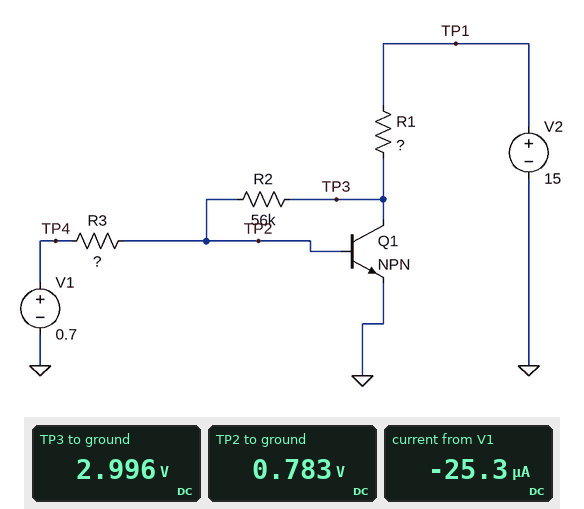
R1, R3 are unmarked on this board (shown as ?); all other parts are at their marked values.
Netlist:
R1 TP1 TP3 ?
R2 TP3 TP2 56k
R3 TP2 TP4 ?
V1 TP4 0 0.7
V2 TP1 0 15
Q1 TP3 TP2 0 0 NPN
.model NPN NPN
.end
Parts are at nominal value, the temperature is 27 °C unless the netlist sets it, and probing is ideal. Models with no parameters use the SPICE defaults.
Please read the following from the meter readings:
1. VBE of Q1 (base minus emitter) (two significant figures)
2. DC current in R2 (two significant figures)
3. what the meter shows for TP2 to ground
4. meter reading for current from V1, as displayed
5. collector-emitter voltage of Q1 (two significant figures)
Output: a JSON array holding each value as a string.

["780 mV", "40 µA", "0.783 V", "-25.3 µA", "3.0 V"]
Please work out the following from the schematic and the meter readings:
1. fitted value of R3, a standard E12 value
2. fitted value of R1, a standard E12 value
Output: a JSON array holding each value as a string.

["3.3 kΩ", "8.2 kΩ"]
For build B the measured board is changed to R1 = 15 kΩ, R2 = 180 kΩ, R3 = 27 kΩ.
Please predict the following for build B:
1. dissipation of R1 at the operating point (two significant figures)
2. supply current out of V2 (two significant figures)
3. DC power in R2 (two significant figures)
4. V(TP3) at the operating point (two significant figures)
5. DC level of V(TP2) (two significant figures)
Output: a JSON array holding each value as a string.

["10 mW", "820 µA", "20 µW", "2.7 V", "770 mV"]
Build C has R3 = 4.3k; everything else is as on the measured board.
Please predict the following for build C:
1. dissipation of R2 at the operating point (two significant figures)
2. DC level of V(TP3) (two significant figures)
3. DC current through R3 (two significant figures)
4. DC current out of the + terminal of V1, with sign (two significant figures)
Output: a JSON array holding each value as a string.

["66 µW", "2.7 V", "20 µA", "-20 µA"]
